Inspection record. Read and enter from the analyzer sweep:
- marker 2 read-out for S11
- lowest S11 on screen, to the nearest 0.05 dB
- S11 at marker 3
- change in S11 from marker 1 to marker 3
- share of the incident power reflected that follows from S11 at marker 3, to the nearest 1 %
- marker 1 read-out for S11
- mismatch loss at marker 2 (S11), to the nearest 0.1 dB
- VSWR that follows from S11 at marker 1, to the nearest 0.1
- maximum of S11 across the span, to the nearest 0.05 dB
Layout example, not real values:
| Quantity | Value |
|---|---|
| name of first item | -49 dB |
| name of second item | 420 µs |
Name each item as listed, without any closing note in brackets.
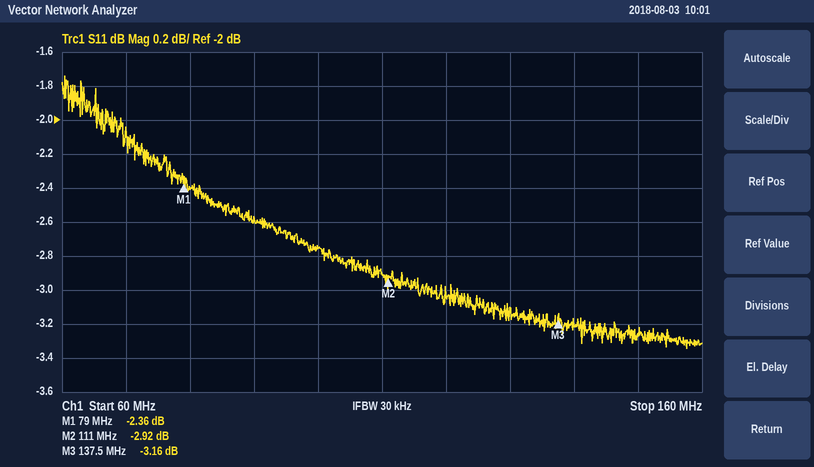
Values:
| Quantity | Value |
|---|---|
| marker 2 read-out for S11 | -2.92 dB |
| lowest S11 on screen, to the nearest 0.05 dB | -3.35 dB |
| S11 at marker 3 | -3.16 dB |
| change in S11 from marker 1 to marker 3 | -0.80 dB |
| share of the incident power reflected that follows from S11 at marker 3, to the nearest 1 % | 48 % |
| marker 1 read-out for S11 | -2.36 dB |
| mismatch loss at marker 2 (S11), to the nearest 0.1 dB | 3.1 dB |
| VSWR that follows from S11 at marker 1, to the nearest 0.1 | 7.4 |
| maximum of S11 across the span, to the nearest 0.05 dB | -1.75 dB |
